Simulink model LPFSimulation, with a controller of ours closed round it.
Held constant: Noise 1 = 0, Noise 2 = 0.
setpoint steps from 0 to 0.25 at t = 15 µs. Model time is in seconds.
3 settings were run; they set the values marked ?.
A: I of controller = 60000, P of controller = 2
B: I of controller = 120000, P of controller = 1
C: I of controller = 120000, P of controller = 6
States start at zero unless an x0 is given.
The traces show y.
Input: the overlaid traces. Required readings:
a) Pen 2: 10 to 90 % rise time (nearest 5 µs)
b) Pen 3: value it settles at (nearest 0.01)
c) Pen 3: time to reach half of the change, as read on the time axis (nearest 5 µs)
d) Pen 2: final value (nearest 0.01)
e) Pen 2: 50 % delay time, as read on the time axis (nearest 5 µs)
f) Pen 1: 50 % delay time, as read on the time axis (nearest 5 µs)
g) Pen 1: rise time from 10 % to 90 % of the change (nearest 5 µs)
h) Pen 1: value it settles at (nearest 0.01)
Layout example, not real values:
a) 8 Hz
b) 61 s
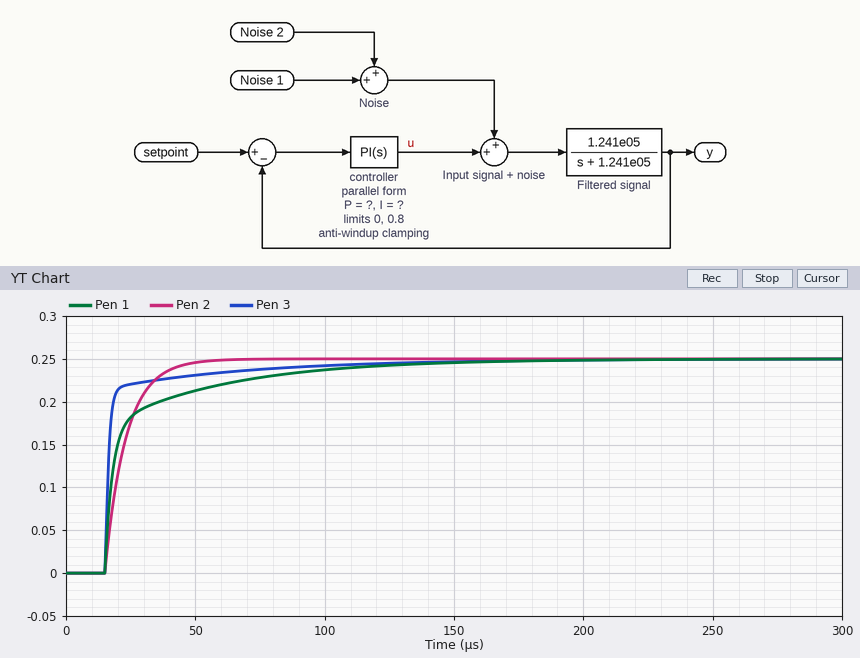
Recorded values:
a) 20 µs
b) 0.25
c) 15 µs
d) 0.25
e) 20 µs
f) 20 µs
g) 55 µs
h) 0.25
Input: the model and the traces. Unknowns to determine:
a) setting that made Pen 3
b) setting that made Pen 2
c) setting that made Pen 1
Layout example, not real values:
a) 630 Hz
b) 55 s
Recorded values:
a) C
b) B
c) A
